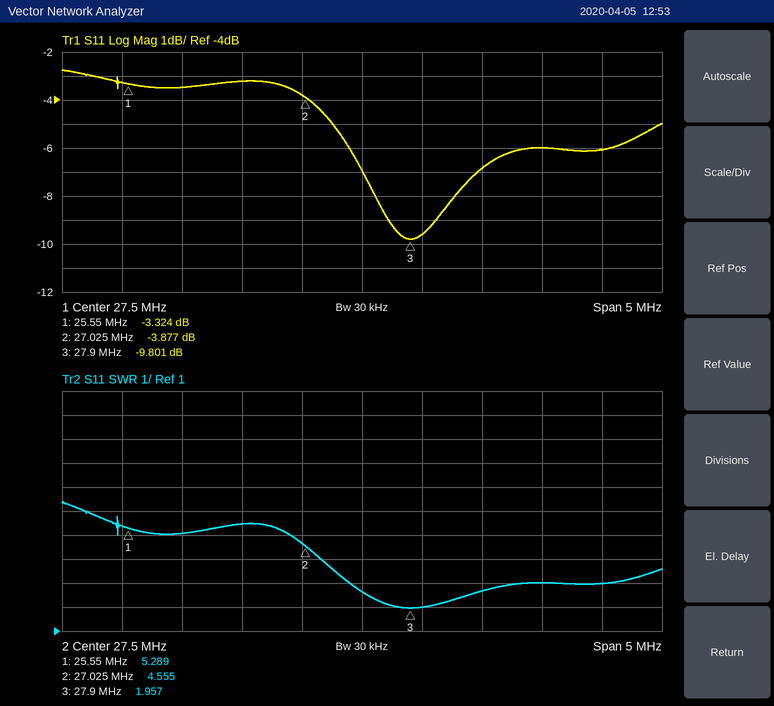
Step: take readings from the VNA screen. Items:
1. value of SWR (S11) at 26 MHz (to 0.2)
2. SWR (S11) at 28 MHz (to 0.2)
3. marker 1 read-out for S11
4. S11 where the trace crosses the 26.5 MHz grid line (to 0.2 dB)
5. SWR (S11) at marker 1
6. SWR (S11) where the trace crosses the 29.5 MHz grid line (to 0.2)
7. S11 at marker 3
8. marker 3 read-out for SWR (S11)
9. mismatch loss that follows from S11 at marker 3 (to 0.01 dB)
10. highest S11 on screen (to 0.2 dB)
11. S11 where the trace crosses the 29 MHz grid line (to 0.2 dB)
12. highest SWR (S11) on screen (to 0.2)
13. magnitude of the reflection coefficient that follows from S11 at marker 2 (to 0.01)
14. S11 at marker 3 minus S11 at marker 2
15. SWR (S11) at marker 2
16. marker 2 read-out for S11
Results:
5.0
2.0
-3.324 dB
-3.2 dB
5.289
3.0
-9.801 dB
1.957
0.48 dB
-2.8 dB
-6.0 dB
6.4
0.64
-5.924 dB
4.555
-3.877 dB
